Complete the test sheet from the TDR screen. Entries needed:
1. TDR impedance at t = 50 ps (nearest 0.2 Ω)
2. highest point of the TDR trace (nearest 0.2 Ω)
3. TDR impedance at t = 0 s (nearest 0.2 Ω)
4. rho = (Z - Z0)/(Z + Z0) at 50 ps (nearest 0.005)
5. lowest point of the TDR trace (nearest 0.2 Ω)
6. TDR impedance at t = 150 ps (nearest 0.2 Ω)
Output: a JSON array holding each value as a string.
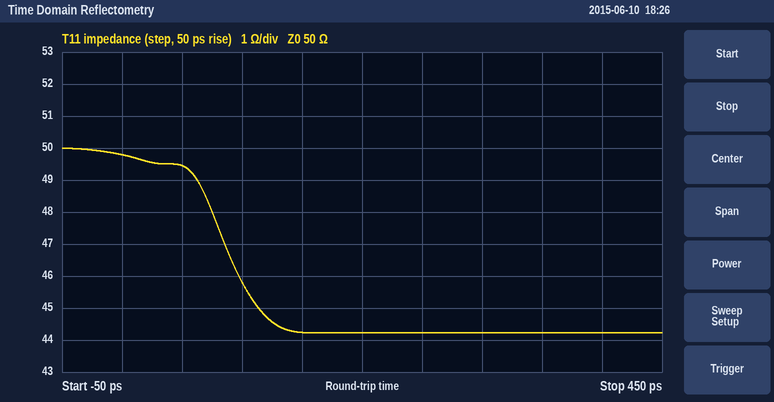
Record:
["49.4 Ω", "50.0 Ω", "49.8 Ω", "-0.005", "44.2 Ω", "44.2 Ω"]
